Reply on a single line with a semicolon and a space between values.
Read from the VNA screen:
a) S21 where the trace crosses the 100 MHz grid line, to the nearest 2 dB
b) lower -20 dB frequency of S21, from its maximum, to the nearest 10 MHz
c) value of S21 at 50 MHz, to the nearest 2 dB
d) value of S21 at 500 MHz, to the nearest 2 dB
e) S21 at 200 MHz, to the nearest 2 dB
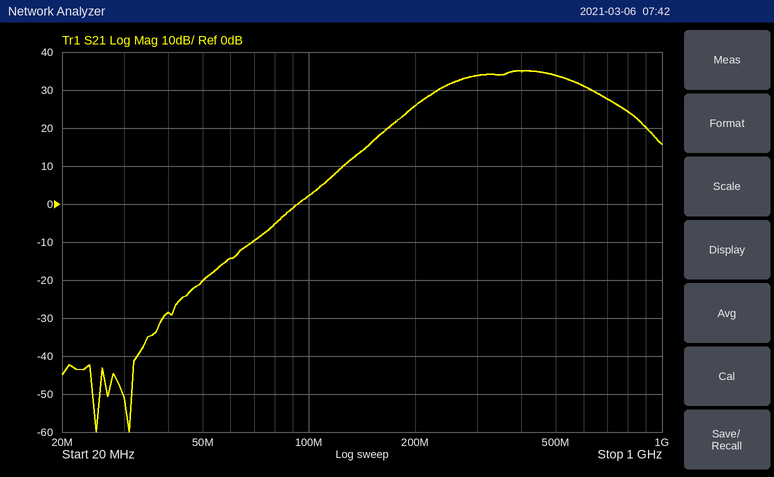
2 dB; 150 MHz; -20 dB; 34 dB; 26 dB
